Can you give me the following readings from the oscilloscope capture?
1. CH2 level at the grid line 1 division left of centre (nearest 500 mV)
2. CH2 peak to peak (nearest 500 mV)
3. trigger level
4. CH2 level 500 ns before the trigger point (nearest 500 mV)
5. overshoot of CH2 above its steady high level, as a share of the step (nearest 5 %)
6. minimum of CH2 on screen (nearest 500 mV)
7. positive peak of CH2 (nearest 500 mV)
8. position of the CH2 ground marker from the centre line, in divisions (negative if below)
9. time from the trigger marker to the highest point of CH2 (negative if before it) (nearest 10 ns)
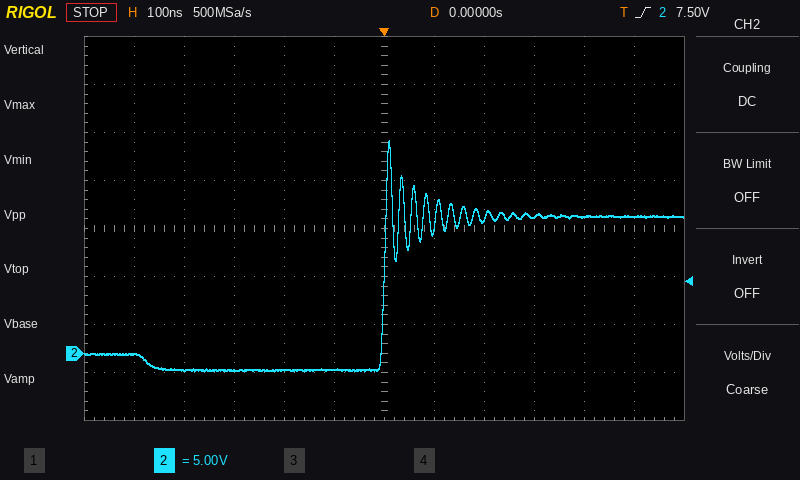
-1.5 V
24.0 V
7.50 V
0.0 V
50 %
-2.0 V
22.0 V
-2.6 div
+10 ns
